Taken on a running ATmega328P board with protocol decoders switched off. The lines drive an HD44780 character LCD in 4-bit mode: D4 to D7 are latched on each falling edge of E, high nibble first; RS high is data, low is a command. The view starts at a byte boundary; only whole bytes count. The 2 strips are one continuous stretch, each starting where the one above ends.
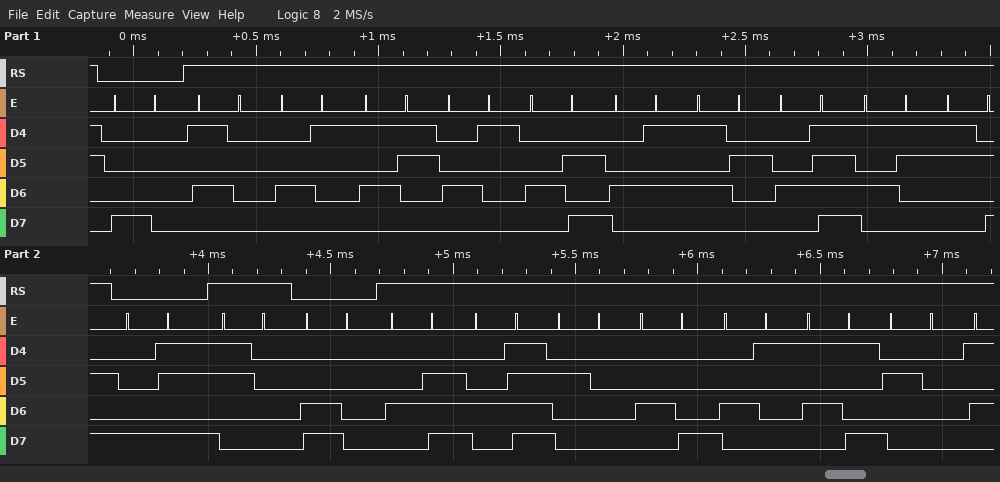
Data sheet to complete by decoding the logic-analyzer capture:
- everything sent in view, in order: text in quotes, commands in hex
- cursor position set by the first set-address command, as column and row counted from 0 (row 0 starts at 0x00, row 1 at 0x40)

0x80 "PASAJEROS:" 0x8B "0" 0xC0 "NO HAY "
column 0, row 0
